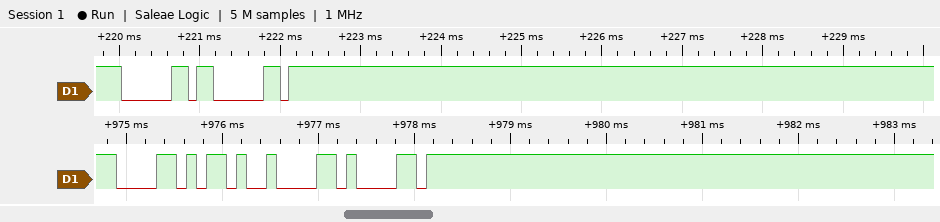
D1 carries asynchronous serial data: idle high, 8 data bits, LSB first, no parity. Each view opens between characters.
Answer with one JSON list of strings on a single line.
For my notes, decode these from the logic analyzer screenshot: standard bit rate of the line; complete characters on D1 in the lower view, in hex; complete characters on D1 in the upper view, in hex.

["9600 baud", "58, 09, 61", "60, 60"]
